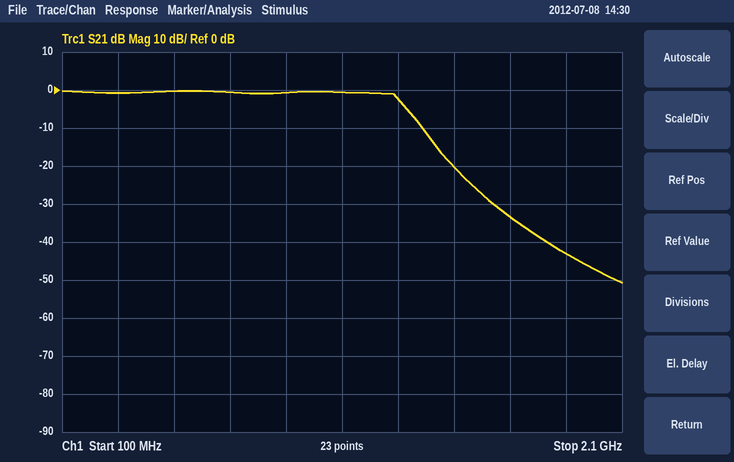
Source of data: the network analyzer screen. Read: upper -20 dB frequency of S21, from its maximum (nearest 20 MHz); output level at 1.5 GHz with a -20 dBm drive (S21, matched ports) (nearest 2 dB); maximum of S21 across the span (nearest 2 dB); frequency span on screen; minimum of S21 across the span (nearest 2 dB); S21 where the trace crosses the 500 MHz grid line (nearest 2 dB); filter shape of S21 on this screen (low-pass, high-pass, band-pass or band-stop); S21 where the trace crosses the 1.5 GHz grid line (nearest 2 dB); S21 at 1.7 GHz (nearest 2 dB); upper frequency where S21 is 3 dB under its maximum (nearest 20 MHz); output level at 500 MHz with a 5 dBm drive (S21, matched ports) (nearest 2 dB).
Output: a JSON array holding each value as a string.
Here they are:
["1.50 GHz", "-40 dBm", "0 dB", "2 GHz", "-50 dB", "0 dB", "low-pass", "-20 dB", "-34 dB", "1.30 GHz", "4 dBm"]
